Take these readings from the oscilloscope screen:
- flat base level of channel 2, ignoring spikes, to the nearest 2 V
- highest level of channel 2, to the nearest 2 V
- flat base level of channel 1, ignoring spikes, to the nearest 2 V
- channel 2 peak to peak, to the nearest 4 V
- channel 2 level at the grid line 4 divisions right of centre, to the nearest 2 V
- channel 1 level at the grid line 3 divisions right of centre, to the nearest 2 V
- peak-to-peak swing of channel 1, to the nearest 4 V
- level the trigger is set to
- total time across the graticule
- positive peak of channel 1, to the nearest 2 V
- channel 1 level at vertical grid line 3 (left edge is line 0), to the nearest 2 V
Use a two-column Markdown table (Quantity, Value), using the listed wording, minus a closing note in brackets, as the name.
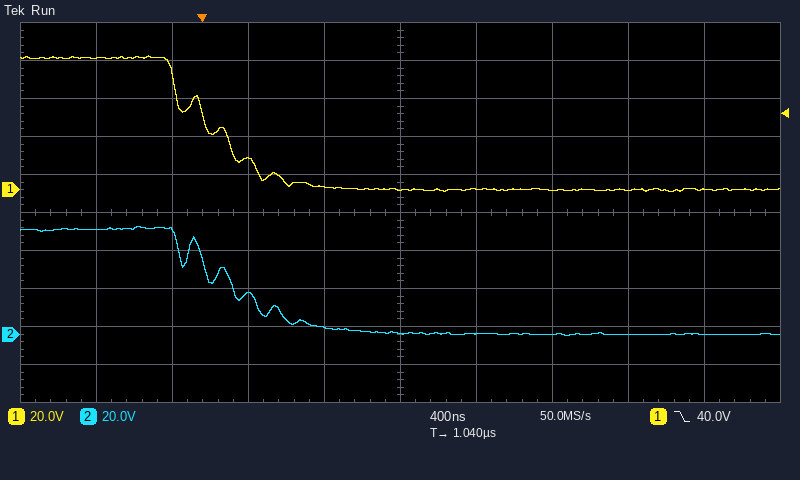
| Quantity | Value |
|---|---|
| flat base level of channel 2, ignoring spikes, to the nearest 2 V | 0 V |
| highest level of channel 2, to the nearest 2 V | 56 V |
| flat base level of channel 1, ignoring spikes, to the nearest 2 V | 0 V |
| channel 2 peak to peak, to the nearest 4 V | 56 V |
| channel 2 level at the grid line 4 divisions right of centre, to the nearest 2 V | 0 V |
| channel 1 level at the grid line 3 divisions right of centre, to the nearest 2 V | 0 V |
| peak-to-peak swing of channel 1, to the nearest 4 V | 72 V |
| level the trigger is set to | 40.0 V |
| total time across the graticule | 4 µs |
| positive peak of channel 1, to the nearest 2 V | 70 V |
| channel 1 level at vertical grid line 3 (left edge is line 0), to the nearest 2 V | 16 V |
